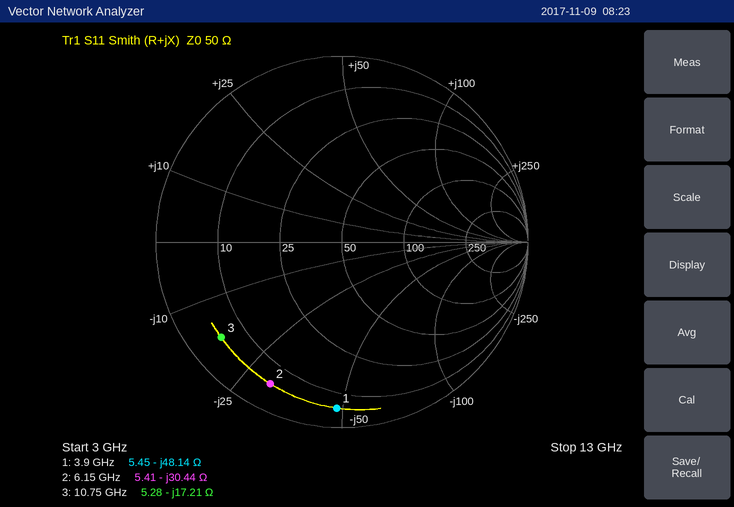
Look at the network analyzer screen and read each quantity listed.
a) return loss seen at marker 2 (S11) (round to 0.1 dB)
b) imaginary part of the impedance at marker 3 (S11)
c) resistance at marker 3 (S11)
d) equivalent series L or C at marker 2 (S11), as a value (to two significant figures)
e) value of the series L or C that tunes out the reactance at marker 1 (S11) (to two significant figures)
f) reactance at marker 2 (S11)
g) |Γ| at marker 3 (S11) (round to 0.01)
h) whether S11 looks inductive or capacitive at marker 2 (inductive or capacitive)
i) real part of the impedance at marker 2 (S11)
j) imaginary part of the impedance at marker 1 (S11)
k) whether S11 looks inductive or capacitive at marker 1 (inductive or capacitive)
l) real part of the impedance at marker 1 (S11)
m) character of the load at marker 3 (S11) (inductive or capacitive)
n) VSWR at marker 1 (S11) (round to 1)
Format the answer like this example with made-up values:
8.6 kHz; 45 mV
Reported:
1.4 dB; -17.21 Ω; 5.28 Ω; 850 fF; 2.0 nH; -30.44 Ω; 0.83; capacitive; 5.41 Ω; -48.14 Ω; capacitive; 5.45 Ω; capacitive; 18
